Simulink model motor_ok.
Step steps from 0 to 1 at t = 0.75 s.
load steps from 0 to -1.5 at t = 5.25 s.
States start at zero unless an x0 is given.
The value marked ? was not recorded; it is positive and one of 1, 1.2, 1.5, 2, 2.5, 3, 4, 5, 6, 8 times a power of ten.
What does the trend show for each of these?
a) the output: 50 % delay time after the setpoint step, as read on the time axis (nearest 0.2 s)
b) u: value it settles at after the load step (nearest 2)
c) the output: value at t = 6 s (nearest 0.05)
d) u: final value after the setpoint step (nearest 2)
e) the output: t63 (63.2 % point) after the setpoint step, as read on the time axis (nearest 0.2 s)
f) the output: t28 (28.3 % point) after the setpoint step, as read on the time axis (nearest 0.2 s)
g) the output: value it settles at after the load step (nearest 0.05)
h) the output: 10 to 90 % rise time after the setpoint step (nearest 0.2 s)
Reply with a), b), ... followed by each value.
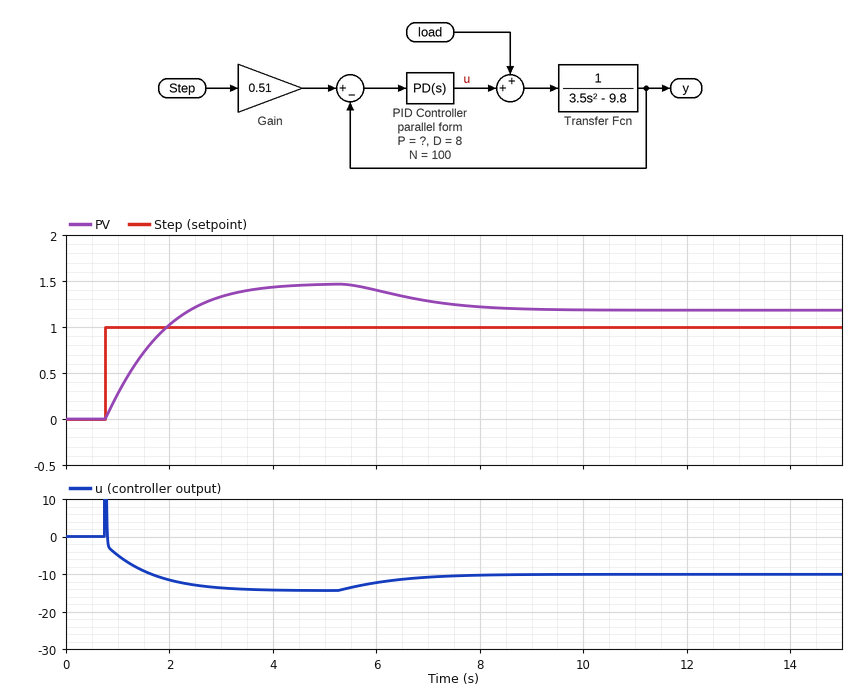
a) 1.6 s
b) -10
c) 1.40
d) -14
e) 1.8 s
f) 1.2 s
g) 1.20
h) 2.0 s
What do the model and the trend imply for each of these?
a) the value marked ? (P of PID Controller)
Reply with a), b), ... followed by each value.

a) 15
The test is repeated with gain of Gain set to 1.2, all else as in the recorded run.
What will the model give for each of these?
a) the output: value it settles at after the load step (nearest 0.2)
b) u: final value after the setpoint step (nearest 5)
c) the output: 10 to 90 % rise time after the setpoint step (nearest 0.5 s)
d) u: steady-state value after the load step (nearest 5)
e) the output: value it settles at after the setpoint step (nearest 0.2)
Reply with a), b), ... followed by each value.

a) 3.2
b) -35
c) 2.0 s
d) -30
e) 3.4
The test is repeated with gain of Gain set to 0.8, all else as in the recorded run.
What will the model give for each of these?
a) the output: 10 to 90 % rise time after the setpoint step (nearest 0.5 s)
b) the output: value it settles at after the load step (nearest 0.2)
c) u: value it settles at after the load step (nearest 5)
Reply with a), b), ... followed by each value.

a) 2.0 s
b) 2.0
c) -20
